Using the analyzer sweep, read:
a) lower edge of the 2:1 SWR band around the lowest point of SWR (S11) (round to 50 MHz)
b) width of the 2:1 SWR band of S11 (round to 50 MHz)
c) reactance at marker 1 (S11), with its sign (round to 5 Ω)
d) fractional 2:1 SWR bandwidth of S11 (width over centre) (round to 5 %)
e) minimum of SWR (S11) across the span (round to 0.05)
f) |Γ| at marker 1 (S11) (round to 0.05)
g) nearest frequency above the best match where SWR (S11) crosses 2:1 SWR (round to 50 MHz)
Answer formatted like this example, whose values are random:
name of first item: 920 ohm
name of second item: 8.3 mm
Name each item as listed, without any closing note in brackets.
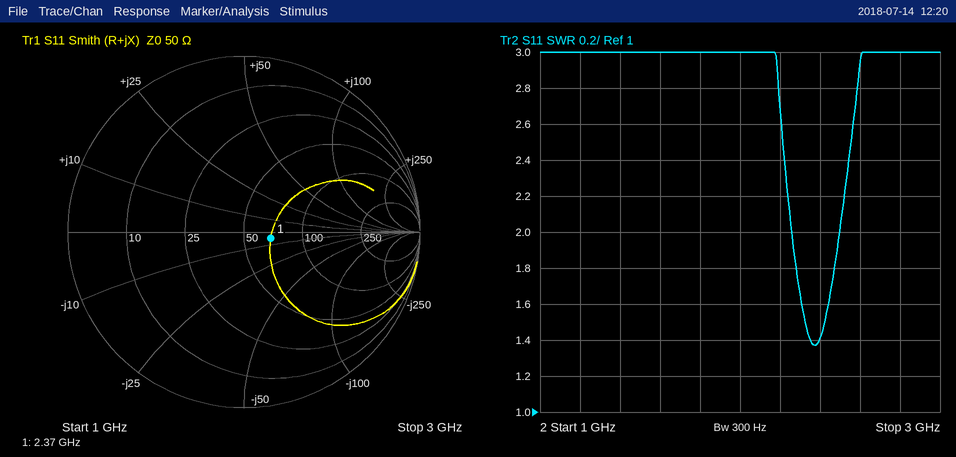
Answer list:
lower edge of the 2:1 SWR band around the lowest point of SWR (S11): 2.25 GHz
width of the 2:1 SWR band of S11: 250 MHz
reactance at marker 1 (S11), with its sign: -5 Ω
fractional 2:1 SWR bandwidth of S11 (width over centre): 10 %
minimum of SWR (S11) across the span: 1.35
|Γ| at marker 1 (S11): 0.15
nearest frequency above the best match where SWR (S11) crosses 2:1 SWR: 2.50 GHz
